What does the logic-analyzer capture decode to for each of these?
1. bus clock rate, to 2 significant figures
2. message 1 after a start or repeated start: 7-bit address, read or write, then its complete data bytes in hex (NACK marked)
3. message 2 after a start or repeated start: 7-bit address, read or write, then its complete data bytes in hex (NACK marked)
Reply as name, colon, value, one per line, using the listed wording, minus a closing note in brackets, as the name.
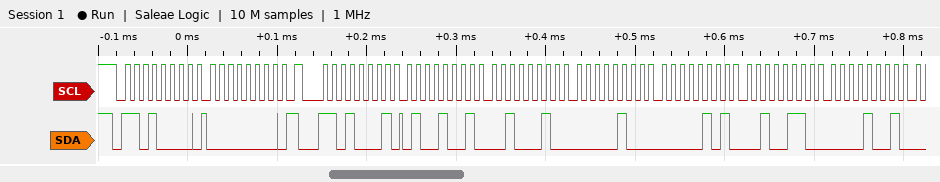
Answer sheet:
bus clock rate, to 2 significant figures: 100 kHz
message 1 after a start or repeated start: 7-bit address, read or write, then its complete data bytes in hex: 0x68 write: 00
message 2 after a start or repeated start: 7-bit address, read or write, then its complete data bytes in hex: 0x68 read: 49 22 04 05 26 09
